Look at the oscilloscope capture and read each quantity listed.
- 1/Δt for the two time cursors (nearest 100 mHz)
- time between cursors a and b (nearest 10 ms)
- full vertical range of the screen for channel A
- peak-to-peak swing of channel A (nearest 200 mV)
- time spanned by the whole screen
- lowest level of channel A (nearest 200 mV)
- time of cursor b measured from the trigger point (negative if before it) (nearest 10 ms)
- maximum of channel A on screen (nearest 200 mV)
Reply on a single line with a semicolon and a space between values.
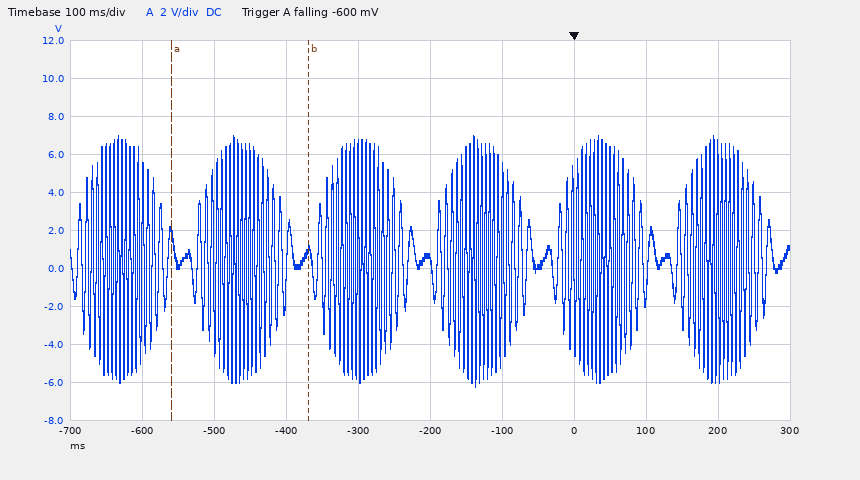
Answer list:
5.3 Hz; 190 ms; 20 V; 13.2 V; 1 s; -6.2 V; -370 ms; 7.0 V
